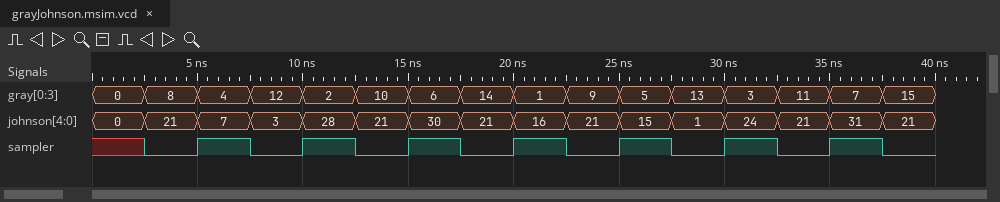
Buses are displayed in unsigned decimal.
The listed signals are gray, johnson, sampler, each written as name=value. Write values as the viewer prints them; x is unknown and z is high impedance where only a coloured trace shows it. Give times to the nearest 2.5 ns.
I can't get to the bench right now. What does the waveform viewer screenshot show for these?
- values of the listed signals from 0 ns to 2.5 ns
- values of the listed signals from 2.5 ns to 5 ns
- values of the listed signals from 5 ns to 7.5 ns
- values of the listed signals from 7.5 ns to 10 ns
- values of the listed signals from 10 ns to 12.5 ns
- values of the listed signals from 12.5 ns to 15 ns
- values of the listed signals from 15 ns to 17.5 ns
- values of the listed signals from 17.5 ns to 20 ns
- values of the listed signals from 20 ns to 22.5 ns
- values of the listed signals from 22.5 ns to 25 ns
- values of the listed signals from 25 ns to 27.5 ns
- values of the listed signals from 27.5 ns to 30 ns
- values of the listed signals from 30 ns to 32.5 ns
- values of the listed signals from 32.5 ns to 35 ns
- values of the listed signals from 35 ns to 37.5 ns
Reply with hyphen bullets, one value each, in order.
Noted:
- gray=0, johnson=0, sampler=x
- gray=8, johnson=21, sampler=0
- gray=4, johnson=7, sampler=1
- gray=12, johnson=3, sampler=0
- gray=2, johnson=28, sampler=1
- gray=10, johnson=21, sampler=0
- gray=6, johnson=30, sampler=1
- gray=14, johnson=21, sampler=0
- gray=1, johnson=16, sampler=1
- gray=9, johnson=21, sampler=0
- gray=5, johnson=15, sampler=1
- gray=13, johnson=1, sampler=0
- gray=3, johnson=24, sampler=1
- gray=11, johnson=21, sampler=0
- gray=7, johnson=31, sampler=1
